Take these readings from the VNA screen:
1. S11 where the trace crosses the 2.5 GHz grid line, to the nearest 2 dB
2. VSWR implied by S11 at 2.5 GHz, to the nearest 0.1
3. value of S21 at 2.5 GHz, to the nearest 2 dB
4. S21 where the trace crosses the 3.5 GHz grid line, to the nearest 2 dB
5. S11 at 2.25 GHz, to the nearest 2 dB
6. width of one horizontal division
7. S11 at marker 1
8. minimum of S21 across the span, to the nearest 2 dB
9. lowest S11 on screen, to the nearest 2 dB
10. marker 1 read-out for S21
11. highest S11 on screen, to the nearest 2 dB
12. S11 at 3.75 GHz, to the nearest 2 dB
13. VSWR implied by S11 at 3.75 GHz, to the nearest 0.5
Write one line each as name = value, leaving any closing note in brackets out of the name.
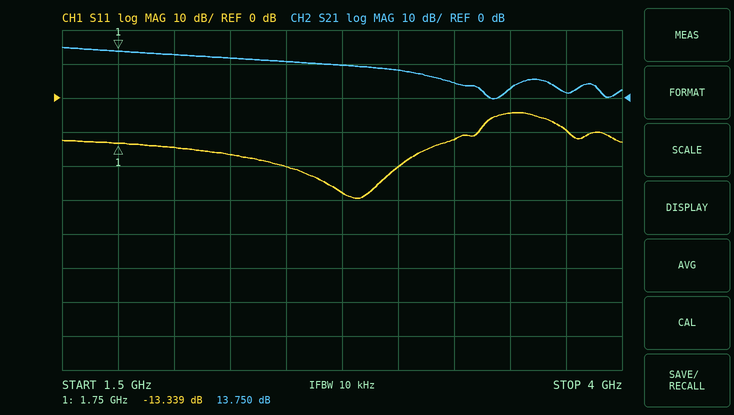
S11 where the trace crosses the 2.5 GHz grid line, to the nearest 2 dB = -20 dB
VSWR implied by S11 at 2.5 GHz, to the nearest 0.1 = 1.2
value of S21 at 2.5 GHz, to the nearest 2 dB = 10 dB
S21 where the trace crosses the 3.5 GHz grid line, to the nearest 2 dB = 2 dB
S11 at 2.25 GHz, to the nearest 2 dB = -16 dB
width of one horizontal division = 250 MHz
S11 at marker 1 = -13.339 dB
minimum of S21 across the span, to the nearest 2 dB = 0 dB
lowest S11 on screen, to the nearest 2 dB = -30 dB
marker 1 read-out for S21 = 13.750 dB
highest S11 on screen, to the nearest 2 dB = -4 dB
S11 at 3.75 GHz, to the nearest 2 dB = -10 dB
VSWR implied by S11 at 3.75 GHz, to the nearest 0.5 = 2.0
